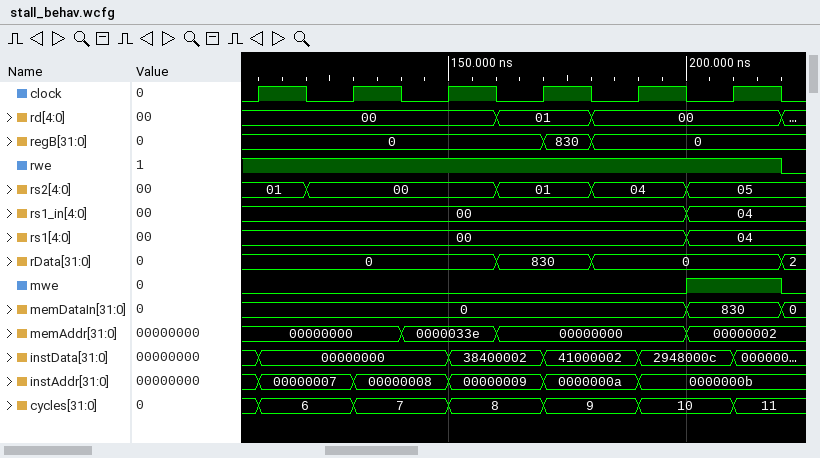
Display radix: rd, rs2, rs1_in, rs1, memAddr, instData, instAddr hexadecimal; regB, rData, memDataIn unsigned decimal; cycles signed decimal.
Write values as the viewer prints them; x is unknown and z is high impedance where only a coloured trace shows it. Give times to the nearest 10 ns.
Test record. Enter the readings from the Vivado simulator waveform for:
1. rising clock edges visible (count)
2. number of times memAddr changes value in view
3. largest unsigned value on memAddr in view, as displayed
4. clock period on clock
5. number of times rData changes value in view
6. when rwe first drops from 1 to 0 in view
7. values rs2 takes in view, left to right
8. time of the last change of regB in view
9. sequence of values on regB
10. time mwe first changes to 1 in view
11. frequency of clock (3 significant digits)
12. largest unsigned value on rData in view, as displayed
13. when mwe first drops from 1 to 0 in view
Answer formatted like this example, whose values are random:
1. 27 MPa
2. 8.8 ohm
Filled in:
1. 6
2. 3
3. 0000033e
4. 20 ns
5. 3
6. 220 ns
7. 01, 00, 01, 04, 05
8. 180 ns
9. 0, 830, 0
10. 200 ns
11. 50.0 MHz
12. 830
13. 220 ns
